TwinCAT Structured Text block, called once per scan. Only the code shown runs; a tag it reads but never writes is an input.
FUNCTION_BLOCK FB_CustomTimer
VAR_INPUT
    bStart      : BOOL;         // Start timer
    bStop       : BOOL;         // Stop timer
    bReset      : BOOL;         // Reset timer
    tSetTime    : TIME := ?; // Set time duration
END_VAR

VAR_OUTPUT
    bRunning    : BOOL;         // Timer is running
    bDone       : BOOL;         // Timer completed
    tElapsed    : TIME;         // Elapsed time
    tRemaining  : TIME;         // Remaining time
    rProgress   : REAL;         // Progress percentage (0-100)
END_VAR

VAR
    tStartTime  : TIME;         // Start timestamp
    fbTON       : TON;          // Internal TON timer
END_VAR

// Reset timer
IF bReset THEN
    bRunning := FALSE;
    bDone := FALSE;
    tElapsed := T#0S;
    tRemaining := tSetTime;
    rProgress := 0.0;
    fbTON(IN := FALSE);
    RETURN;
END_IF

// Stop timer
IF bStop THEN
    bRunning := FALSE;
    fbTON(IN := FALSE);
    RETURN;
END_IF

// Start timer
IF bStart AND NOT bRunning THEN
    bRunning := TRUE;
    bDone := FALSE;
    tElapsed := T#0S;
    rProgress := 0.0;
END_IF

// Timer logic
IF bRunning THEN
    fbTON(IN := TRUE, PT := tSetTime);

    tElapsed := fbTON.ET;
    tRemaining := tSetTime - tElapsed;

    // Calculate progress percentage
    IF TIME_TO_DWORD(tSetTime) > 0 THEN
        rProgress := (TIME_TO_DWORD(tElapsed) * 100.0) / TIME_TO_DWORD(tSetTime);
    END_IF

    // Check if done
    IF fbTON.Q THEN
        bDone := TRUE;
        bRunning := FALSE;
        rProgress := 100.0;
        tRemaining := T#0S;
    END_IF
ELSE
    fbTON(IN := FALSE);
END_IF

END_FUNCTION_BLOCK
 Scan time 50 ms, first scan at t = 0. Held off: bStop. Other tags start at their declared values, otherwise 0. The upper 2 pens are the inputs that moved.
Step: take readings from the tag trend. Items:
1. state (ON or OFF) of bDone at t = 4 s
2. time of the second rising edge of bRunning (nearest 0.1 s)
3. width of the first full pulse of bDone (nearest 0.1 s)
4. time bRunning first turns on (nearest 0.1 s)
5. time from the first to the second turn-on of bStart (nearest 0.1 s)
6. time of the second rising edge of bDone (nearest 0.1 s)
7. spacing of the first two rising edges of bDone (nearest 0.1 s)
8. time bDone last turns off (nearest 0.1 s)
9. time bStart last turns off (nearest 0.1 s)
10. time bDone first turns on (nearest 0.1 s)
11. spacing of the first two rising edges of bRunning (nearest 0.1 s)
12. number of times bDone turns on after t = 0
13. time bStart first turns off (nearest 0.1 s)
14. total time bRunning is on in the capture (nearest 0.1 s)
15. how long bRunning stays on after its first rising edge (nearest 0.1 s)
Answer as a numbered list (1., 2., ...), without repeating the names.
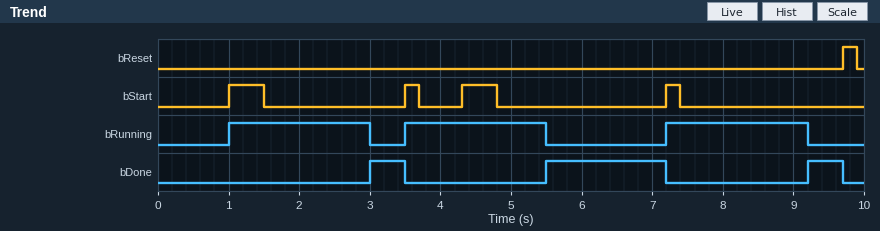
1. OFF
2. 3.5 s
3. 0.5 s
4. 1.0 s
5. 2.5 s
6. 5.5 s
7. 2.5 s
8. 9.7 s
9. 7.4 s
10. 3.0 s
11. 2.5 s
12. 3
13. 1.5 s
14. 6.0 s
15. 2.0 s
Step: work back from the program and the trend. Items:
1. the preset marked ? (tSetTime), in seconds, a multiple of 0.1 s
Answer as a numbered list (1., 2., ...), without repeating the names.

1. 2.0 s
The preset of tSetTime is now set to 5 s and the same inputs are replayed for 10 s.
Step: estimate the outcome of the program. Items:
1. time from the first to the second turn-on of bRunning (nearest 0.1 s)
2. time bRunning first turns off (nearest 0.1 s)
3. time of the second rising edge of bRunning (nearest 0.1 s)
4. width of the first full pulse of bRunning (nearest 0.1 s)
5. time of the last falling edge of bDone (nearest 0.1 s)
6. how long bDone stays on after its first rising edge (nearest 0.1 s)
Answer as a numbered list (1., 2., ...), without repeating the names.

1. 6.2 s
2. 6.0 s
3. 7.2 s
4. 5.0 s
5. 7.2 s
6. 1.2 s
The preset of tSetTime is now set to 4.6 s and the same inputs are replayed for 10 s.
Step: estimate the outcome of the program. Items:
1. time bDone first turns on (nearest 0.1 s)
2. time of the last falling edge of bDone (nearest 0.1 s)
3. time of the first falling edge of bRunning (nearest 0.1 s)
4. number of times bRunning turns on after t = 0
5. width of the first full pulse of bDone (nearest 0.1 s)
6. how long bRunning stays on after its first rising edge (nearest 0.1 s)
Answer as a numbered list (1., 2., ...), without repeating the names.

1. 5.6 s
2. 7.2 s
3. 5.6 s
4. 2
5. 1.6 s
6. 4.6 s
